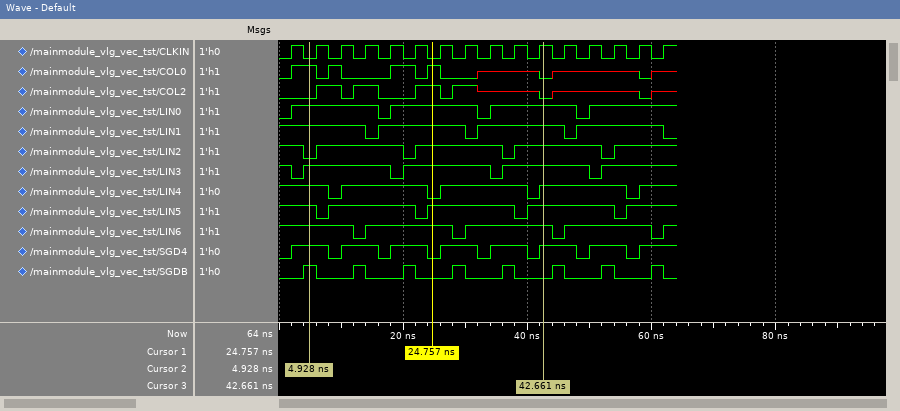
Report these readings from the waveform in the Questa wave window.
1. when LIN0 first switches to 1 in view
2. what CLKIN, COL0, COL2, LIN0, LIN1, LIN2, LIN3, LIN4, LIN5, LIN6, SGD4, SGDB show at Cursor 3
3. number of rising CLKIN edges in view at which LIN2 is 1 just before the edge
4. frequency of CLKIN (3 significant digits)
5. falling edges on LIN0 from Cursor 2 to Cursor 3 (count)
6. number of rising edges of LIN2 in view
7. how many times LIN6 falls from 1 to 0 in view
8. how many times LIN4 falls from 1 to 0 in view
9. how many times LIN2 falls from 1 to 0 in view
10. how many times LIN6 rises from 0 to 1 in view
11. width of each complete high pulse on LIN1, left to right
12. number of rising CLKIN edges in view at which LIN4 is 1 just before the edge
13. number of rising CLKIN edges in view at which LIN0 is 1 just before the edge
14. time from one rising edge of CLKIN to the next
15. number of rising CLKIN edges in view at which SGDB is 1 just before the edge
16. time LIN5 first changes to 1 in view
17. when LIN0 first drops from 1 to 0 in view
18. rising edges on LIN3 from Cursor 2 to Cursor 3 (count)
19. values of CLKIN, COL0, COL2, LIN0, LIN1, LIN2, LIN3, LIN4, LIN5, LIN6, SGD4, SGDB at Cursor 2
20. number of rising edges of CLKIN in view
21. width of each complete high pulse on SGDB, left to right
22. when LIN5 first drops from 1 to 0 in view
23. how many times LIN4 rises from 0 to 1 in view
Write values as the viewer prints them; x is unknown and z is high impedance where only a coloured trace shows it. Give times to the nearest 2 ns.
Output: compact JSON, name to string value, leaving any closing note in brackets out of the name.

{"when LIN0 first switches to 1 in view": "2 ns", "what CLKIN, COL0, COL2, LIN0, LIN1, LIN2, LIN3, LIN4, LIN5, LIN6, SGD4, SGDB show at Cursor 3": "CLKIN=1, COL0=0, COL2=0, LIN0=1, LIN1=1, LIN2=1, LIN3=1, LIN4=1, LIN5=1, LIN6=1, SGD4=1, SGDB=0", "number of rising CLKIN edges in view at which LIN2 is 1 just before the edge": "12", "frequency of CLKIN": "250 MHz", "falling edges on LIN0 from Cursor 2 to Cursor 3": "2", "number of rising edges of LIN2 in view": "4", "how many times LIN6 falls from 1 to 0 in view": "4", "how many times LIN4 falls from 1 to 0 in view": "4", "how many times LIN2 falls from 1 to 0 in view": "4", "how many times LIN6 rises from 0 to 1 in view": "4", "width of each complete high pulse on LIN1, left to right": "14 ns, 14 ns, 14 ns", "number of rising CLKIN edges in view at which LIN4 is 1 just before the edge": "12", "number of rising CLKIN edges in view at which LIN0 is 1 just before the edge": "12", "time from one rising edge of CLKIN to the next": "4 ns", "number of rising CLKIN edges in view at which SGDB is 1 just before the edge": "8", "time LIN5 first changes to 1 in view": "8 ns", "when LIN0 first drops from 1 to 0 in view": "16 ns", "rising edges on LIN3 from Cursor 2 to Cursor 3": "2", "values of CLKIN, COL0, COL2, LIN0, LIN1, LIN2, LIN3, LIN4, LIN5, LIN6, SGD4, SGDB at Cursor 2": "CLKIN=0, COL0=1, COL2=0, LIN0=1, LIN1=1, LIN2=0, LIN3=1, LIN4=1, LIN5=1, LIN6=1, SGD4=1, SGDB=1", "number of rising edges of CLKIN in view": "16", "width of each complete high pulse on SGDB, left to right": "2 ns, 2 ns, 2 ns, 2 ns, 2 ns, 2 ns, 2 ns, 2 ns", "when LIN5 first drops from 1 to 0 in view": "6 ns", "how many times LIN4 rises from 0 to 1 in view": "4"}
